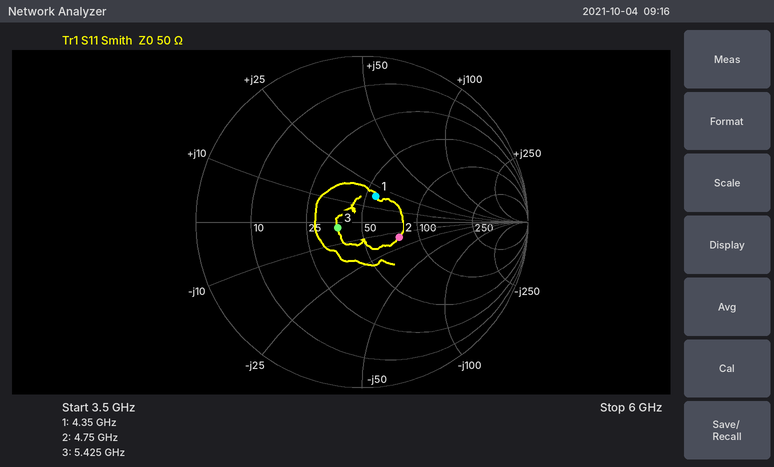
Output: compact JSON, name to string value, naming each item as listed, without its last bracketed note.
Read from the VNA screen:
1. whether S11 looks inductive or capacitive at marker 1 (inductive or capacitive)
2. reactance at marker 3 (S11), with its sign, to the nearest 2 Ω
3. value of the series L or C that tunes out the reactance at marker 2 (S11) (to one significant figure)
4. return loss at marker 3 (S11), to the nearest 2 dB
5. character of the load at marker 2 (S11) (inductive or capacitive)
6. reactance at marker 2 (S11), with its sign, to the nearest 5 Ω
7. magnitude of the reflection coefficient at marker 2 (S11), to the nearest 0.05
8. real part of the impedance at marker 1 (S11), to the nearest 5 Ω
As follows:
{"whether S11 looks inductive or capacitive at marker 1": "inductive", "reactance at marker 3 (S11), with its sign, to the nearest 2 Ω": "-2 Ω", "value of the series L or C that tunes out the reactance at marker 2 (S11)": "500 pH", "return loss at marker 3 (S11), to the nearest 2 dB": "16 dB", "character of the load at marker 2 (S11)": "capacitive", "reactance at marker 2 (S11), with its sign, to the nearest 5 Ω": "-15 Ω", "magnitude of the reflection coefficient at marker 2 (S11), to the nearest 0.05": "0.25", "real part of the impedance at marker 1 (S11), to the nearest 5 Ω": "55 Ω"}
